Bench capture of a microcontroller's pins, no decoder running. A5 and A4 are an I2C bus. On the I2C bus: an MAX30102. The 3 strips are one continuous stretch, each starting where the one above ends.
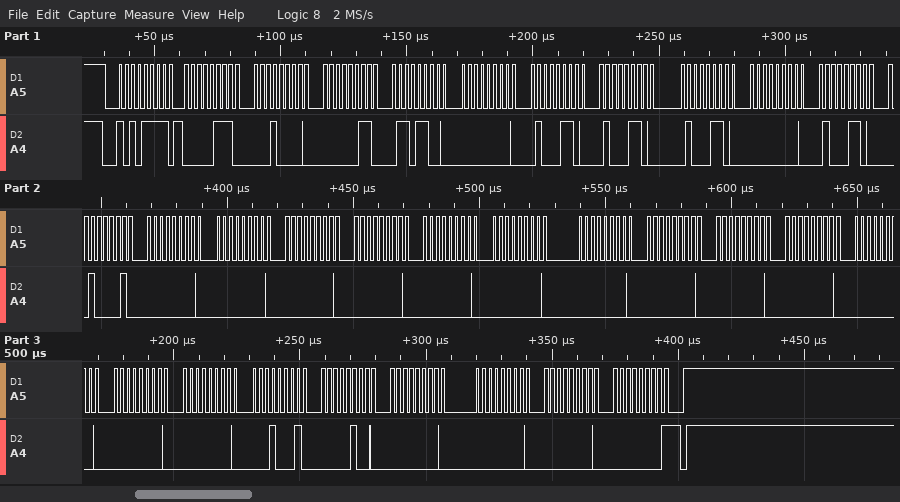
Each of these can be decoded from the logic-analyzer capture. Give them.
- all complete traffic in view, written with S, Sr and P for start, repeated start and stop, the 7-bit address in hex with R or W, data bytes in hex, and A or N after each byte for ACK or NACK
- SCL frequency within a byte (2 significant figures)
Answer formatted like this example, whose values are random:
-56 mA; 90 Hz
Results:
S 57R A 07 A 10 A 03 A 6C A 00 A 46 A 46 A 46 A 00 A 46 A 21 A 00 A 00 A 00 A 00 A 00 A 00 A 00 A 00 A 00 A 00 A 00 A 00 A 00 A 11 A 04 A 00 A 00 A 00 A 00 N P; 400 kHz
